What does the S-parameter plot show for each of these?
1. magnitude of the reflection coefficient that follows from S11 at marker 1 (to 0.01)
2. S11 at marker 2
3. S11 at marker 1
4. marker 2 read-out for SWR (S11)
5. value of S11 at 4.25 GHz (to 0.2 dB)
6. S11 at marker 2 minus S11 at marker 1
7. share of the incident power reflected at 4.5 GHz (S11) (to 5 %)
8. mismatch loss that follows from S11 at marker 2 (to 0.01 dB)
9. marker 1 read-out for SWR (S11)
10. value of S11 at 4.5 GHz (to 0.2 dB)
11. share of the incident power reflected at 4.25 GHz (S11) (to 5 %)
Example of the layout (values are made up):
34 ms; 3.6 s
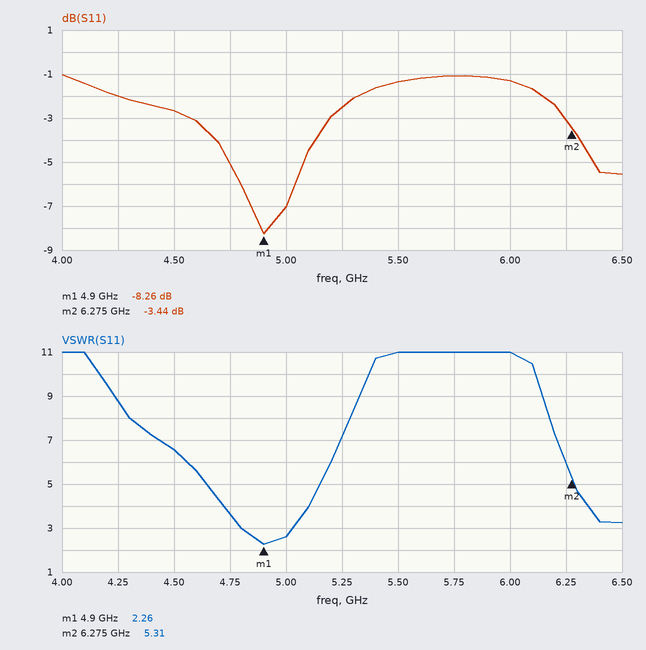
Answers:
0.39; -3.44 dB; -8.26 dB; 5.31; -2.0 dB; 4.82 dB; 55 %; 2.62 dB; 2.26; -2.6 dB; 65 %
